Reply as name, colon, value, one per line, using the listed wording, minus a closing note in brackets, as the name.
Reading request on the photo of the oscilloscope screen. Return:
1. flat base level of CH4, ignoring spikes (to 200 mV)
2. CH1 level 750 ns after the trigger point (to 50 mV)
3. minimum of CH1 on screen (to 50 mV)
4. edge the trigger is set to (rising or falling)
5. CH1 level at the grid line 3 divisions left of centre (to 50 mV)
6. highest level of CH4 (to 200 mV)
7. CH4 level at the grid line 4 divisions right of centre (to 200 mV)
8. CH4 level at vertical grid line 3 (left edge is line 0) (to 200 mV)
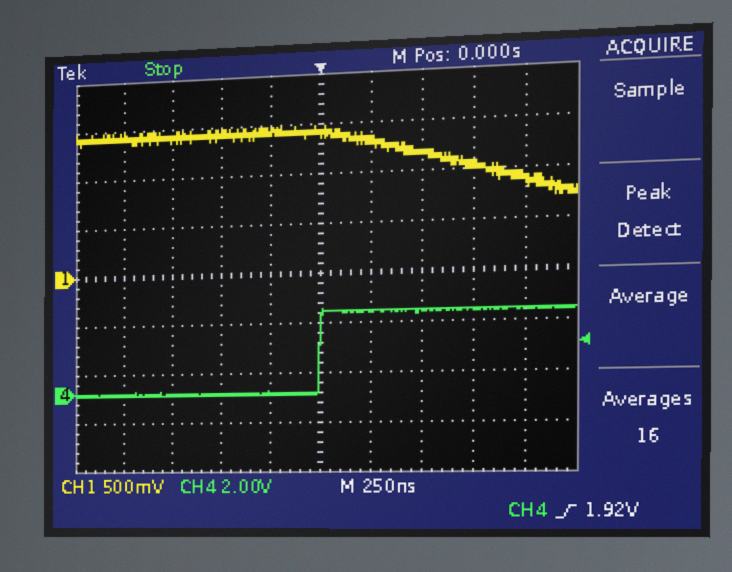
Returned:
flat base level of CH4, ignoring spikes: 0.0 V
CH1 level 750 ns after the trigger point: 1.05 V
minimum of CH1 on screen: 700 mV
edge the trigger is set to: rising
CH1 level at the grid line 3 divisions left of centre: 1.40 V
highest level of CH4: 3.4 V
CH4 level at the grid line 4 divisions right of centre: 3.2 V
CH4 level at vertical grid line 3 (left edge is line 0): 0.0 V
